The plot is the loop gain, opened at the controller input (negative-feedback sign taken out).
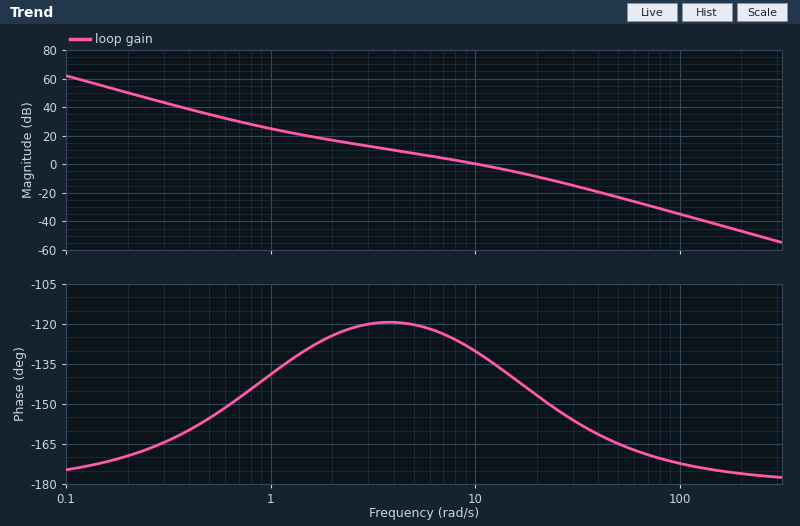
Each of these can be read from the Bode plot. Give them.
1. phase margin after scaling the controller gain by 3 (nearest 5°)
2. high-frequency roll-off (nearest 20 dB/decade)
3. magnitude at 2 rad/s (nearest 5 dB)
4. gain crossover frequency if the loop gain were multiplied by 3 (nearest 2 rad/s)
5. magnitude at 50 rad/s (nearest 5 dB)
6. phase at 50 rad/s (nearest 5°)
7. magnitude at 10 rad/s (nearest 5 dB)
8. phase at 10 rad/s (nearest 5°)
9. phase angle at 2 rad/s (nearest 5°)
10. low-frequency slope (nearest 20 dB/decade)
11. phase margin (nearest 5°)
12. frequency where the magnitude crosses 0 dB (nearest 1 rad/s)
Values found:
30°
-40 dB/decade
15 dB
22 rad/s
-25 dB
-165°
0 dB
-130°
-125°
-40 dB/decade
50°
10 rad/s
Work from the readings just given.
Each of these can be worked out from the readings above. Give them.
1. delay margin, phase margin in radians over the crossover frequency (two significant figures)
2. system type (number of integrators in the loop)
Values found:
0.087 s
2
